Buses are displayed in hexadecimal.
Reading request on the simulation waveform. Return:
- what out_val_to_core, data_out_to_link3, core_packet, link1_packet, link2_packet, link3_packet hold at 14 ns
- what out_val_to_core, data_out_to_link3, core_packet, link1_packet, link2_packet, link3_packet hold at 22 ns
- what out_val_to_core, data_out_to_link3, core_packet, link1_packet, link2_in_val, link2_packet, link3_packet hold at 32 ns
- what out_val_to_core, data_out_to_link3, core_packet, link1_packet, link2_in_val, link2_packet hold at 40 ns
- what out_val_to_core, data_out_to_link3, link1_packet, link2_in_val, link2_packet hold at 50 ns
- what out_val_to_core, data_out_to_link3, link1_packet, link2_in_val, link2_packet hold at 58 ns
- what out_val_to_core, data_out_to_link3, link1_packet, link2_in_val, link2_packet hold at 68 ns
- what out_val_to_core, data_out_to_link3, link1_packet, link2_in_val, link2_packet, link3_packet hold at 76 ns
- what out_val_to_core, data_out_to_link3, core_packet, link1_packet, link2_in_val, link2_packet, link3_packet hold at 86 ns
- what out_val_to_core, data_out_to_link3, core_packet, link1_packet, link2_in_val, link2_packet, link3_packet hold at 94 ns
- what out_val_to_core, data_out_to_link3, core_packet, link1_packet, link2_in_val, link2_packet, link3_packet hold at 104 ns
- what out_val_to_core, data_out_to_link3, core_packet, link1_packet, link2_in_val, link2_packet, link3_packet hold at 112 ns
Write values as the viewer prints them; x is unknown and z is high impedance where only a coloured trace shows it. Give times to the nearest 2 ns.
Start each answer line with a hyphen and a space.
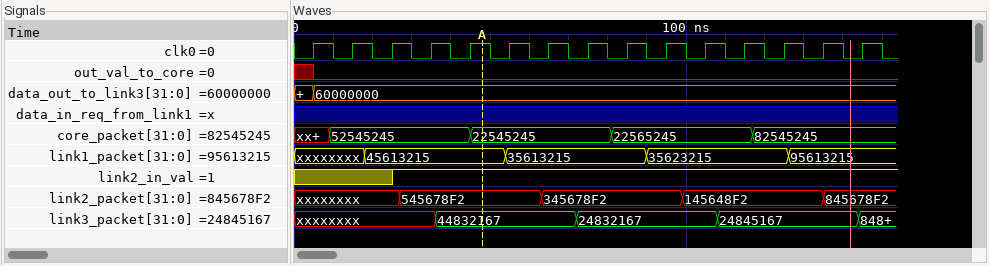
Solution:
- out_val_to_core=0, data_out_to_link3=60000000, core_packet=52545245, link1_packet=xxxxxxxx, link2_packet=xxxxxxxx, link3_packet=xxxxxxxx
- out_val_to_core=0, data_out_to_link3=60000000, core_packet=52545245, link1_packet=45613215, link2_packet=xxxxxxxx, link3_packet=xxxxxxxx
- out_val_to_core=0, data_out_to_link3=60000000, core_packet=52545245, link1_packet=45613215, link2_in_val=1, link2_packet=545678F2, link3_packet=xxxxxxxx
- out_val_to_core=0, data_out_to_link3=60000000, core_packet=52545245, link1_packet=45613215, link2_in_val=1, link2_packet=545678F2
- out_val_to_core=0, data_out_to_link3=60000000, link1_packet=45613215, link2_in_val=1, link2_packet=545678F2
- out_val_to_core=0, data_out_to_link3=60000000, link1_packet=35613215, link2_in_val=1, link2_packet=545678F2
- out_val_to_core=0, data_out_to_link3=60000000, link1_packet=35613215, link2_in_val=1, link2_packet=345678F2
- out_val_to_core=0, data_out_to_link3=60000000, link1_packet=35613215, link2_in_val=1, link2_packet=345678F2, link3_packet=24832167
- out_val_to_core=0, data_out_to_link3=60000000, core_packet=22565245, link1_packet=35613215, link2_in_val=1, link2_packet=345678F2, link3_packet=24832167
- out_val_to_core=0, data_out_to_link3=60000000, core_packet=22565245, link1_packet=35623215, link2_in_val=1, link2_packet=345678F2, link3_packet=24832167
- out_val_to_core=0, data_out_to_link3=60000000, core_packet=22565245, link1_packet=35623215, link2_in_val=1, link2_packet=145648F2, link3_packet=24832167
- out_val_to_core=0, data_out_to_link3=60000000, core_packet=22565245, link1_packet=35623215, link2_in_val=1, link2_packet=145648F2, link3_packet=24845167
